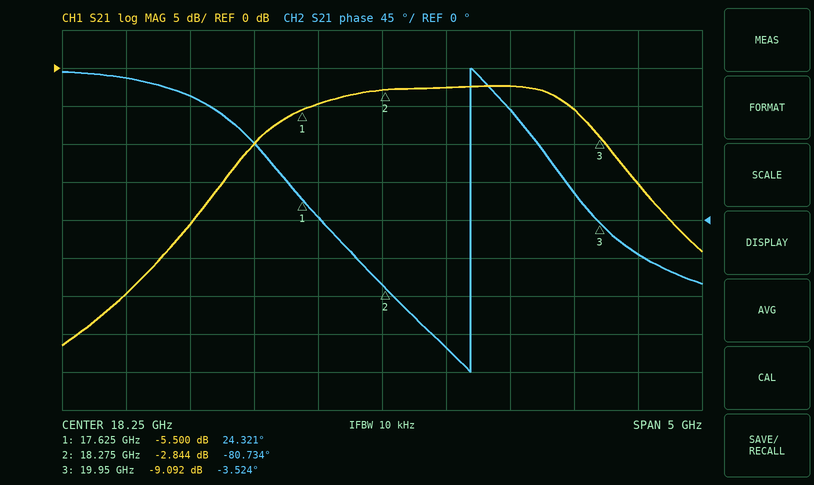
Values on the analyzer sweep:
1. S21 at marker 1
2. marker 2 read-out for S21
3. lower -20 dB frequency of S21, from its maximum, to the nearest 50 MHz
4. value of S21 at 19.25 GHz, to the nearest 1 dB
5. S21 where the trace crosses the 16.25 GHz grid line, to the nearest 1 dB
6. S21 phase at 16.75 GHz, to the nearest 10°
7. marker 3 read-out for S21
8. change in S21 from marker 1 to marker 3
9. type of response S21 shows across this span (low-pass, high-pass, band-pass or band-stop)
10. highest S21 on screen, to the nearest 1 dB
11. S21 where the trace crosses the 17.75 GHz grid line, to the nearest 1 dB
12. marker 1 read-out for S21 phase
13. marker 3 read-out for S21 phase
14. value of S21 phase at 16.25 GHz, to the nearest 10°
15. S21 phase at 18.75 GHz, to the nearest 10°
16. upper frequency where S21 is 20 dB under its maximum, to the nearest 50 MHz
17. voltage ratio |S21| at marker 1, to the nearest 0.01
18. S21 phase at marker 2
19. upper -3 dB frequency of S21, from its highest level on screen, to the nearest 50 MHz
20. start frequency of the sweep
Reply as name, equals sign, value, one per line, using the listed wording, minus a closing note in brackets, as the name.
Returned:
S21 at marker 1 = -5.500 dB
marker 2 read-out for S21 = -2.844 dB
lower -20 dB frequency of S21, from its maximum, to the nearest 50 MHz = 16.65 GHz
value of S21 at 19.25 GHz, to the nearest 1 dB = -2 dB
S21 where the trace crosses the 16.25 GHz grid line, to the nearest 1 dB = -30 dB
S21 phase at 16.75 GHz, to the nearest 10° = 150°
marker 3 read-out for S21 = -9.092 dB
change in S21 from marker 1 to marker 3 = -3.592 dB
type of response S21 shows across this span = band-pass
highest S21 on screen, to the nearest 1 dB = -2 dB
S21 where the trace crosses the 17.75 GHz grid line, to the nearest 1 dB = -5 dB
marker 1 read-out for S21 phase = 24.321°
marker 3 read-out for S21 phase = -3.524°
value of S21 phase at 16.25 GHz, to the nearest 10° = 170°
S21 phase at 18.75 GHz, to the nearest 10° = -150°
upper frequency where S21 is 20 dB under its maximum, to the nearest 50 MHz = 20.65 GHz
voltage ratio |S21| at marker 1, to the nearest 0.01 = 0.53
S21 phase at marker 2 = -80.734°
upper -3 dB frequency of S21, from its highest level on screen, to the nearest 50 MHz = 19.75 GHz
start frequency of the sweep = 15.75 GHz
